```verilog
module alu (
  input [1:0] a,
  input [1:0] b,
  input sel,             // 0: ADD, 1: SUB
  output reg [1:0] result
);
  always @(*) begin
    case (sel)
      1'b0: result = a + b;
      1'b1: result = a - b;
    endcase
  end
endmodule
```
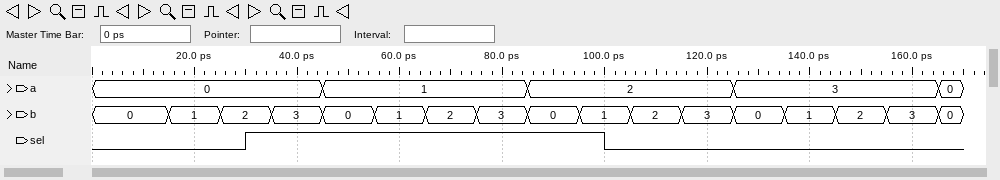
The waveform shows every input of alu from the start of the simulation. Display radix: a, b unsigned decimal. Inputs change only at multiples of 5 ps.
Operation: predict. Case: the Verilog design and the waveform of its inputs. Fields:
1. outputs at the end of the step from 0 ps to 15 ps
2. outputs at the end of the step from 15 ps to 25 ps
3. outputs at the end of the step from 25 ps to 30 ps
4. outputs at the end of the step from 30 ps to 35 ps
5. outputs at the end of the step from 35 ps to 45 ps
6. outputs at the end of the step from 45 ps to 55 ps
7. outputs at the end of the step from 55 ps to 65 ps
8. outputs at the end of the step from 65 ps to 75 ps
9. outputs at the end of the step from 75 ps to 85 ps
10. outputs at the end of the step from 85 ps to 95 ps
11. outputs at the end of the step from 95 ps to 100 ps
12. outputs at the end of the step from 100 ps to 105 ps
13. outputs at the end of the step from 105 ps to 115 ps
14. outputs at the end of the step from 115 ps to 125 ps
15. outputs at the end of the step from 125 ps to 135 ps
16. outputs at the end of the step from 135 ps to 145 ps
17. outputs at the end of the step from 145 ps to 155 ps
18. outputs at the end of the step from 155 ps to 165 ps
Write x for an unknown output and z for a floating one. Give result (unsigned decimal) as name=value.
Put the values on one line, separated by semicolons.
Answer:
result=0; result=1; result=2; result=2; result=1; result=1; result=0; result=3; result=2; result=2; result=1; result=3; result=0; result=1; result=3; result=0; result=1; result=2
